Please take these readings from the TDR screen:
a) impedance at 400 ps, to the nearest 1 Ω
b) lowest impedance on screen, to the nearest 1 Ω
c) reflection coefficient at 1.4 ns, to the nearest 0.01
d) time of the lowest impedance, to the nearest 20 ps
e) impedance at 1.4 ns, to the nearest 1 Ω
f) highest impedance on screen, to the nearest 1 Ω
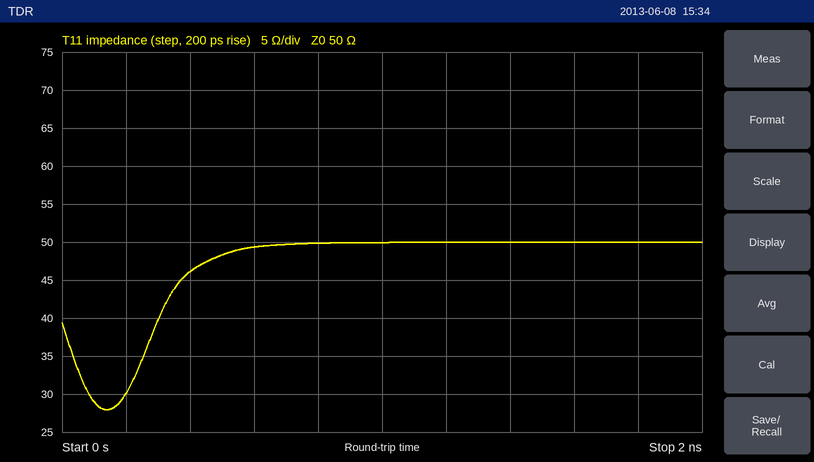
46 Ω
28 Ω
0.00
140 ps
50 Ω
50 Ω
